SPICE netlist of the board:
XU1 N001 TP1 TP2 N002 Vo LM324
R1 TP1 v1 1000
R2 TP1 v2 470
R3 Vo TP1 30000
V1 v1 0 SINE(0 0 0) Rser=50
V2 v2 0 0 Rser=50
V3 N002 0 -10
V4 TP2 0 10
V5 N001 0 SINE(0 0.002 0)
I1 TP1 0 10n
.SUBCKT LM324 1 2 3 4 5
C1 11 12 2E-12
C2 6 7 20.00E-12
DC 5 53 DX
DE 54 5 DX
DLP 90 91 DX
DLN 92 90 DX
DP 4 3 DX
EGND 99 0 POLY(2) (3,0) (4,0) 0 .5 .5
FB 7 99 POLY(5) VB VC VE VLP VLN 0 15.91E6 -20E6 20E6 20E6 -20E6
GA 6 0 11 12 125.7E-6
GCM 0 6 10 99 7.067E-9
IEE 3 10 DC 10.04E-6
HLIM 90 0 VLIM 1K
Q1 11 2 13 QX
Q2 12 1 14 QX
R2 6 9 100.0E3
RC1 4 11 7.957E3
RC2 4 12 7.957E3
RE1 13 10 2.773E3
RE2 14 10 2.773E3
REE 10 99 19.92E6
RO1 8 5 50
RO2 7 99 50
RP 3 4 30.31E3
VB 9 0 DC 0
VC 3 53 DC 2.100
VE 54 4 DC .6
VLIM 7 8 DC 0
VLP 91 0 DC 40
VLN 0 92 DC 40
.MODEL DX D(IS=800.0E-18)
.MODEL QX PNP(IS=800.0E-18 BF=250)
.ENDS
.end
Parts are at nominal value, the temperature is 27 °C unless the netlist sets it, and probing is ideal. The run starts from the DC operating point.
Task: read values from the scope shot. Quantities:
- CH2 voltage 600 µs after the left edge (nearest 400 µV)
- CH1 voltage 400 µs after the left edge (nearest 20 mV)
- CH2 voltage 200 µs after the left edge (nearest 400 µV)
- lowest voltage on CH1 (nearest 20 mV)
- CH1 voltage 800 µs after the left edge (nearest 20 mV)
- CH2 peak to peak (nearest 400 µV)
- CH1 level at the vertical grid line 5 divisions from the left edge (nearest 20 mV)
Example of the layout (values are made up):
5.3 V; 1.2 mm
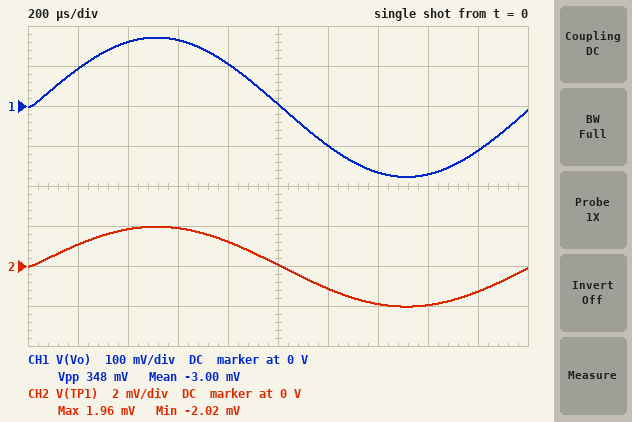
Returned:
2.0 mV; 160 mV; 1.2 mV; -180 mV; 100 mV; 4.0 mV; 0 V
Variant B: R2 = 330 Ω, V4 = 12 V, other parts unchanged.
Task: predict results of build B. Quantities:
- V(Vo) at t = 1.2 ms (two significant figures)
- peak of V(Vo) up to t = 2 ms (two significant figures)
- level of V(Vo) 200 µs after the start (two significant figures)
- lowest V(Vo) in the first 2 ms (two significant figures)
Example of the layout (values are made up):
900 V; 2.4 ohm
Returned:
-110 mV; 220 mV; 120 mV; -210 mV
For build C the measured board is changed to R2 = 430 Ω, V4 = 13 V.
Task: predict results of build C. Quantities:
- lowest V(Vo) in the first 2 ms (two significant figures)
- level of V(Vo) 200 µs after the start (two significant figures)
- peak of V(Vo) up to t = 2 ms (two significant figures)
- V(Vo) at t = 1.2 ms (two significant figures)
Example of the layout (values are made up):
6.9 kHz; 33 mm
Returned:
-180 mV; 110 mV; 190 mV; -95 mV
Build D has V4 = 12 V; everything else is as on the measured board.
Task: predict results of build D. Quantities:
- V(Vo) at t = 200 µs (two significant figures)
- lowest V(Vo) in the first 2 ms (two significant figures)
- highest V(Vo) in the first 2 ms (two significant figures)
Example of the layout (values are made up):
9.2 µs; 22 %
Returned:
99 mV; -170 mV; 180 mV
